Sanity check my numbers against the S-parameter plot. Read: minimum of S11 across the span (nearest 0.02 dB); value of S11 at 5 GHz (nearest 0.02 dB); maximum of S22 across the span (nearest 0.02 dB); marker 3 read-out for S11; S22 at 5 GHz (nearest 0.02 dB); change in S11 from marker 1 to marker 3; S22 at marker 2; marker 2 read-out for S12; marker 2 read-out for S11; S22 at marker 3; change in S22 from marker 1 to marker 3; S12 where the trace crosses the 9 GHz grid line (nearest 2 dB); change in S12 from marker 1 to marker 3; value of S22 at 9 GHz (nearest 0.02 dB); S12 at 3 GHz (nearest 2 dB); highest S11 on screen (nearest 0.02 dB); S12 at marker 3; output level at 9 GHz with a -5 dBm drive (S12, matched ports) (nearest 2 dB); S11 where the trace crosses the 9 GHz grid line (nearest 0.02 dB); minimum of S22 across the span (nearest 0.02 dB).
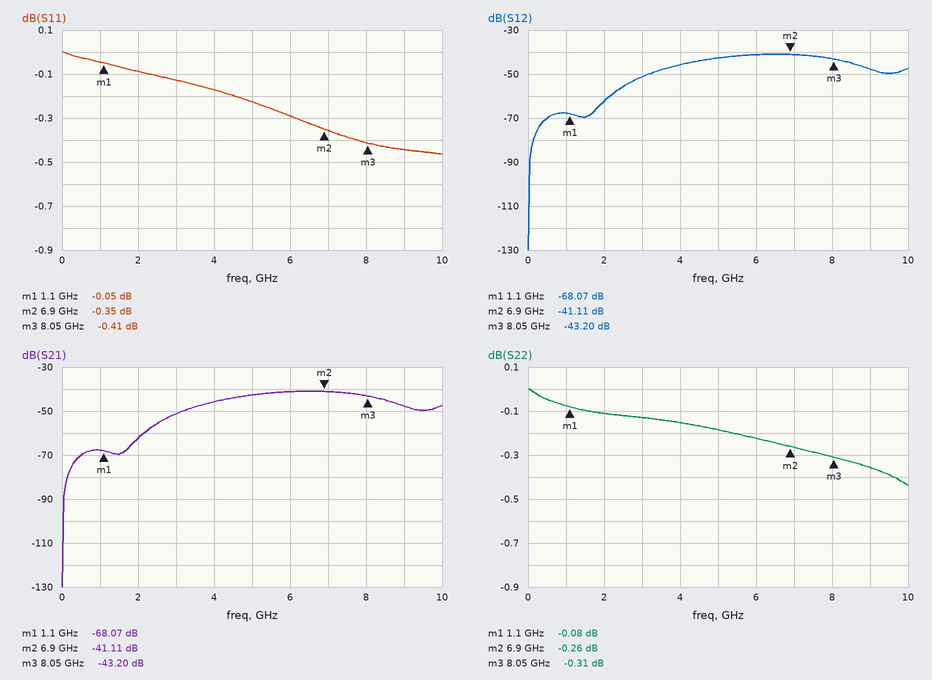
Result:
-0.46 dB
-0.22 dB
0.00 dB
-0.41 dB
-0.18 dB
-0.36 dB
-0.26 dB
-41.11 dB
-0.35 dB
-0.31 dB
-0.23 dB
-48 dB
24.87 dB
-0.36 dB
-52 dB
0.00 dB
-43.20 dB
-52 dBm
-0.44 dB
-0.44 dB
